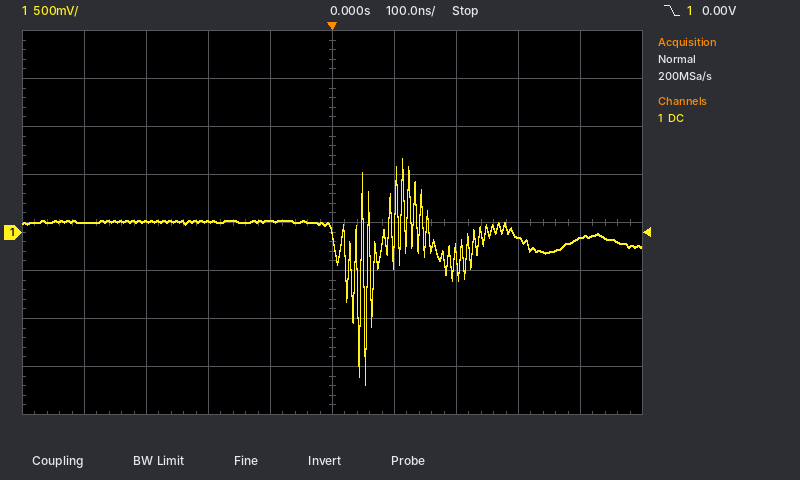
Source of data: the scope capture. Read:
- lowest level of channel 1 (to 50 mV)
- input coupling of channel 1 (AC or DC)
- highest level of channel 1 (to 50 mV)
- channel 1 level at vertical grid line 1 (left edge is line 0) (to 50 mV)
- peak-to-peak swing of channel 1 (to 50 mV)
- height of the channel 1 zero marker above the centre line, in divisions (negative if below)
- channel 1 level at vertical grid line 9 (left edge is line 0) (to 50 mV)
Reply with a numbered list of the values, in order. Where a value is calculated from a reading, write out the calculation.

1. -1.60 V
2. DC
3. 750 mV
4. 100 mV
5. 750 mV − (-1.60 V) = 2.35 V
6. -0.2 div
7. -50 mV
